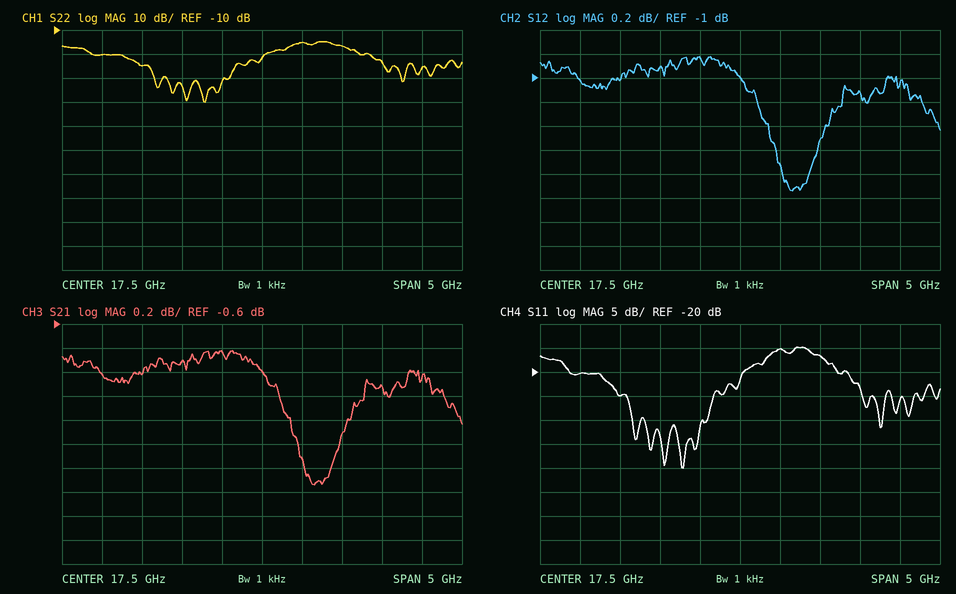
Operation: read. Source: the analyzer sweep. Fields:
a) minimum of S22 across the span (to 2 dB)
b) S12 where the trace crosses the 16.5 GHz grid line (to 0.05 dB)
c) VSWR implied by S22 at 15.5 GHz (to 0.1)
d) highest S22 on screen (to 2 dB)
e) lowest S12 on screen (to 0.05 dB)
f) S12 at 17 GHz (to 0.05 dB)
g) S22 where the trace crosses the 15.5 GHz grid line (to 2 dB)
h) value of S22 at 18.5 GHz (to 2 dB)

-40 dB
-0.90 dB
1.2
-14 dB
-1.95 dB
-0.85 dB
-20 dB
-16 dB
